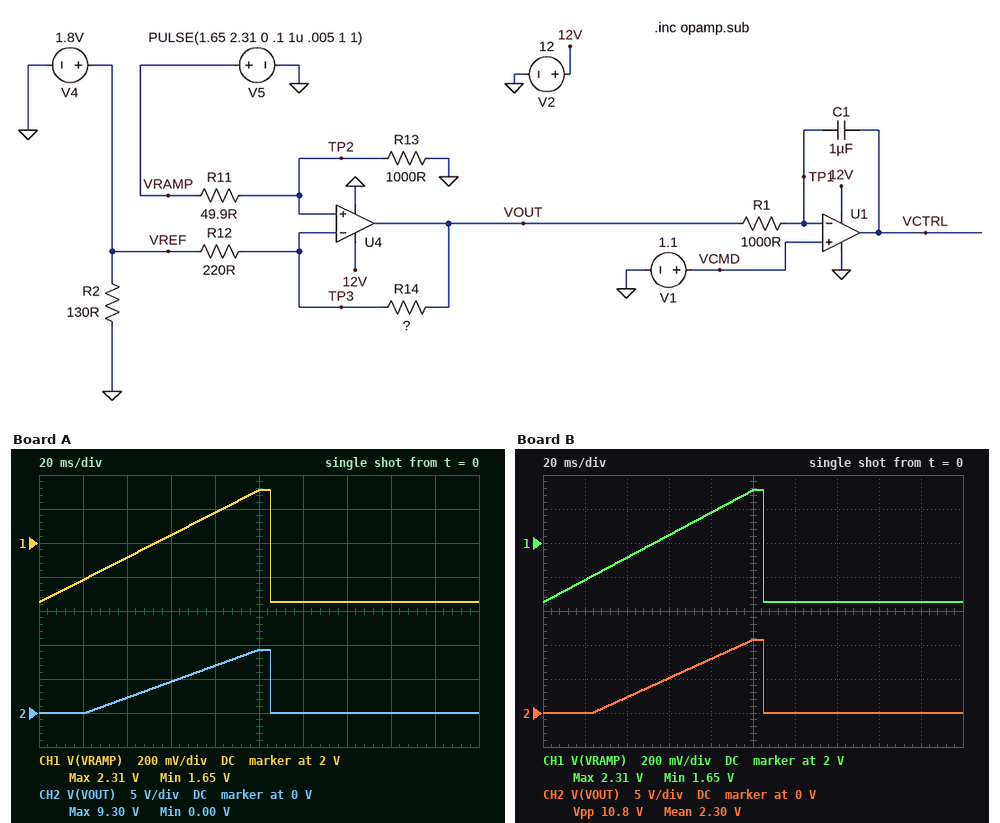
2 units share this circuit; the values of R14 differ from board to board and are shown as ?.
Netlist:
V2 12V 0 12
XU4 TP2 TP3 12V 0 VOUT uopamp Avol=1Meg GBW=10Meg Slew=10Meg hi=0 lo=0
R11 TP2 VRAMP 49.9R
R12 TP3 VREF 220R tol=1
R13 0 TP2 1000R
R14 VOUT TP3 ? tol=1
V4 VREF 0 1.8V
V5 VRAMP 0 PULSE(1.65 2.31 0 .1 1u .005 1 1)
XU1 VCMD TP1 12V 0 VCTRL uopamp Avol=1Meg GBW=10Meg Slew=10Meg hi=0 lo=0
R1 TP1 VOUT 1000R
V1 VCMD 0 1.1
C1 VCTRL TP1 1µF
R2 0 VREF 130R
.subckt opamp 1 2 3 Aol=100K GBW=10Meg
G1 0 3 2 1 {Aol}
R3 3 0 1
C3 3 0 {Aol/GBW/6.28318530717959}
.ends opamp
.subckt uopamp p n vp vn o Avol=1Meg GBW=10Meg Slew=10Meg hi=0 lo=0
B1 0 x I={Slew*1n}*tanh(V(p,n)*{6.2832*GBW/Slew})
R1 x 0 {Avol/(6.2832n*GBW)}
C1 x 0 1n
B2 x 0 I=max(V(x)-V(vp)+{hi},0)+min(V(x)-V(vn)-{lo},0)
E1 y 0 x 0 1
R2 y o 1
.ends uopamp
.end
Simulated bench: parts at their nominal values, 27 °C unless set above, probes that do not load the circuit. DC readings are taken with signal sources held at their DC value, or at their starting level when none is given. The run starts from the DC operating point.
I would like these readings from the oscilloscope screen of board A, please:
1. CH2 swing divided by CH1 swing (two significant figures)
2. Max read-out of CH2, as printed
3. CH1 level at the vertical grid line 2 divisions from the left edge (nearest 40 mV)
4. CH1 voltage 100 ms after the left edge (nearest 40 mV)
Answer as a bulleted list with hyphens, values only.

- 14
- 9.30 V
- 1.92 V
- 2.32 V
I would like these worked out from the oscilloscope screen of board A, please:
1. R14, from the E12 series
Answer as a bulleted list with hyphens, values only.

- 3.9 kΩ
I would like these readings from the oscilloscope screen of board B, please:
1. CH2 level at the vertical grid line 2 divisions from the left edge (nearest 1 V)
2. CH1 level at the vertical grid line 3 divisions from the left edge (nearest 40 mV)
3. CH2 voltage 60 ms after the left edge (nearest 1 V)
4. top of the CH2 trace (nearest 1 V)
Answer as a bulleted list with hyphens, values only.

- 2 V
- 2.04 V
- 5 V
- 11 V
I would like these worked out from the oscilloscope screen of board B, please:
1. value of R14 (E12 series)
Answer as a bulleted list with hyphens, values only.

- 4.7 kΩ
